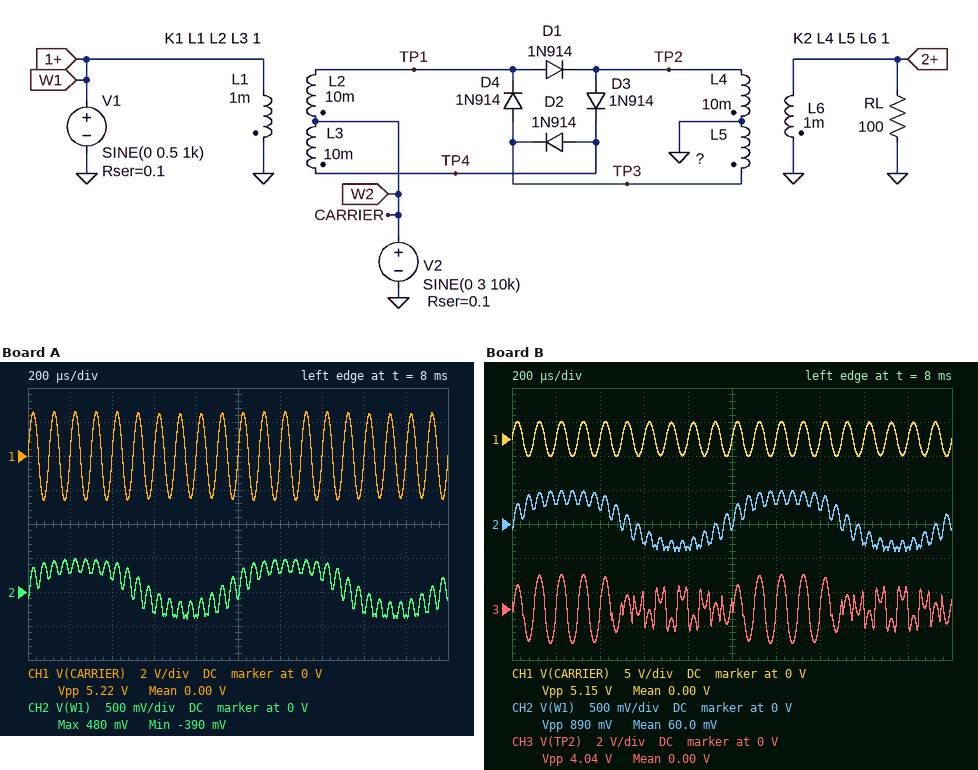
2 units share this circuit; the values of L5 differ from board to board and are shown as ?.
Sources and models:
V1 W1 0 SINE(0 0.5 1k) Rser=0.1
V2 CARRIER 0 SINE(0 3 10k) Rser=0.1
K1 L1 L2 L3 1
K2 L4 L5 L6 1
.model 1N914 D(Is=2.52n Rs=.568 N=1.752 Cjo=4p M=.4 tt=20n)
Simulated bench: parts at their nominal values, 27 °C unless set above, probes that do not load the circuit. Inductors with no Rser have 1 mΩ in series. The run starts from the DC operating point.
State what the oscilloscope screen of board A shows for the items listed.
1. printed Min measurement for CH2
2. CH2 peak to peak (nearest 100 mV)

-390 mV
900 mV
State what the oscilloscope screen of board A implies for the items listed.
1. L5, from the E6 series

3.3 mH
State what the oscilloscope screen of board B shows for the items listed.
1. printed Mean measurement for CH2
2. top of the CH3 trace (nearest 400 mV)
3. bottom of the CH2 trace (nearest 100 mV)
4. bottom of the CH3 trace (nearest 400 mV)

60.0 mV
2.0 V
-400 mV
-2.0 V
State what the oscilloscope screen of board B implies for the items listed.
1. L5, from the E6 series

4.7 mH
